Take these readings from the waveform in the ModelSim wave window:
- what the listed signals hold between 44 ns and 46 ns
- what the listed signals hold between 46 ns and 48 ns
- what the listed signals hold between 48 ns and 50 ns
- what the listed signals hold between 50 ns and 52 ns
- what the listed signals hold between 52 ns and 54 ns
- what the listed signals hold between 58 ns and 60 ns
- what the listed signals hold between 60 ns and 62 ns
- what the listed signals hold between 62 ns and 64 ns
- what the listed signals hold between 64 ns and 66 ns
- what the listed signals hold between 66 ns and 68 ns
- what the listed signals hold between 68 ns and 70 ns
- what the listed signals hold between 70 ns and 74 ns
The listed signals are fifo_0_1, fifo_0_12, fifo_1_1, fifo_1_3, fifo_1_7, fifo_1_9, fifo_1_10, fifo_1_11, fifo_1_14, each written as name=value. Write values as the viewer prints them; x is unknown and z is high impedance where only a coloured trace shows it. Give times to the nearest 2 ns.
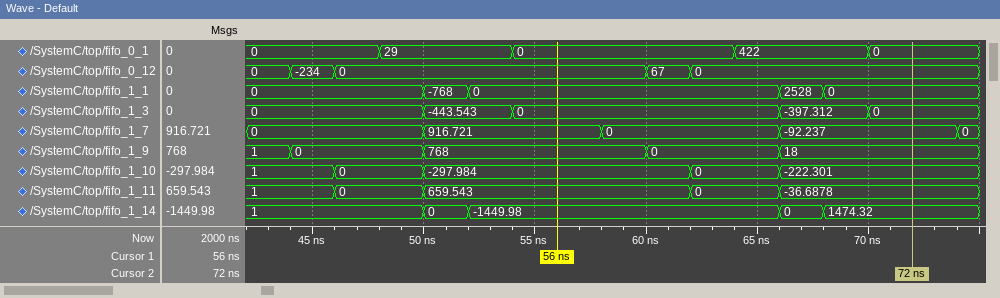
fifo_0_1=0, fifo_0_12=-234, fifo_1_1=0, fifo_1_3=0, fifo_1_7=0, fifo_1_9=0, fifo_1_10=1, fifo_1_11=1, fifo_1_14=1
fifo_0_1=0, fifo_0_12=0, fifo_1_1=0, fifo_1_3=0, fifo_1_7=0, fifo_1_9=0, fifo_1_10=0, fifo_1_11=0, fifo_1_14=1
fifo_0_1=29, fifo_0_12=0, fifo_1_1=0, fifo_1_3=0, fifo_1_7=0, fifo_1_9=0, fifo_1_10=0, fifo_1_11=0, fifo_1_14=1
fifo_0_1=29, fifo_0_12=0, fifo_1_1=-768, fifo_1_3=-443.543, fifo_1_7=916.721, fifo_1_9=768, fifo_1_10=-297.984, fifo_1_11=659.543, fifo_1_14=0
fifo_0_1=29, fifo_0_12=0, fifo_1_1=0, fifo_1_3=-443.543, fifo_1_7=916.721, fifo_1_9=768, fifo_1_10=-297.984, fifo_1_11=659.543, fifo_1_14=-1449.98
fifo_0_1=0, fifo_0_12=0, fifo_1_1=0, fifo_1_3=0, fifo_1_7=0, fifo_1_9=768, fifo_1_10=-297.984, fifo_1_11=659.543, fifo_1_14=-1449.98
fifo_0_1=0, fifo_0_12=67, fifo_1_1=0, fifo_1_3=0, fifo_1_7=0, fifo_1_9=0, fifo_1_10=-297.984, fifo_1_11=659.543, fifo_1_14=-1449.98
fifo_0_1=0, fifo_0_12=0, fifo_1_1=0, fifo_1_3=0, fifo_1_7=0, fifo_1_9=0, fifo_1_10=0, fifo_1_11=0, fifo_1_14=-1449.98
fifo_0_1=422, fifo_0_12=0, fifo_1_1=0, fifo_1_3=0, fifo_1_7=0, fifo_1_9=0, fifo_1_10=0, fifo_1_11=0, fifo_1_14=-1449.98
fifo_0_1=422, fifo_0_12=0, fifo_1_1=2528, fifo_1_3=-397.312, fifo_1_7=-92.237, fifo_1_9=18, fifo_1_10=-222.301, fifo_1_11=-36.6878, fifo_1_14=0
fifo_0_1=422, fifo_0_12=0, fifo_1_1=0, fifo_1_3=-397.312, fifo_1_7=-92.237, fifo_1_9=18, fifo_1_10=-222.301, fifo_1_11=-36.6878, fifo_1_14=1474.32
fifo_0_1=0, fifo_0_12=0, fifo_1_1=0, fifo_1_3=0, fifo_1_7=-92.237, fifo_1_9=18, fifo_1_10=-222.301, fifo_1_11=-36.6878, fifo_1_14=1474.32
